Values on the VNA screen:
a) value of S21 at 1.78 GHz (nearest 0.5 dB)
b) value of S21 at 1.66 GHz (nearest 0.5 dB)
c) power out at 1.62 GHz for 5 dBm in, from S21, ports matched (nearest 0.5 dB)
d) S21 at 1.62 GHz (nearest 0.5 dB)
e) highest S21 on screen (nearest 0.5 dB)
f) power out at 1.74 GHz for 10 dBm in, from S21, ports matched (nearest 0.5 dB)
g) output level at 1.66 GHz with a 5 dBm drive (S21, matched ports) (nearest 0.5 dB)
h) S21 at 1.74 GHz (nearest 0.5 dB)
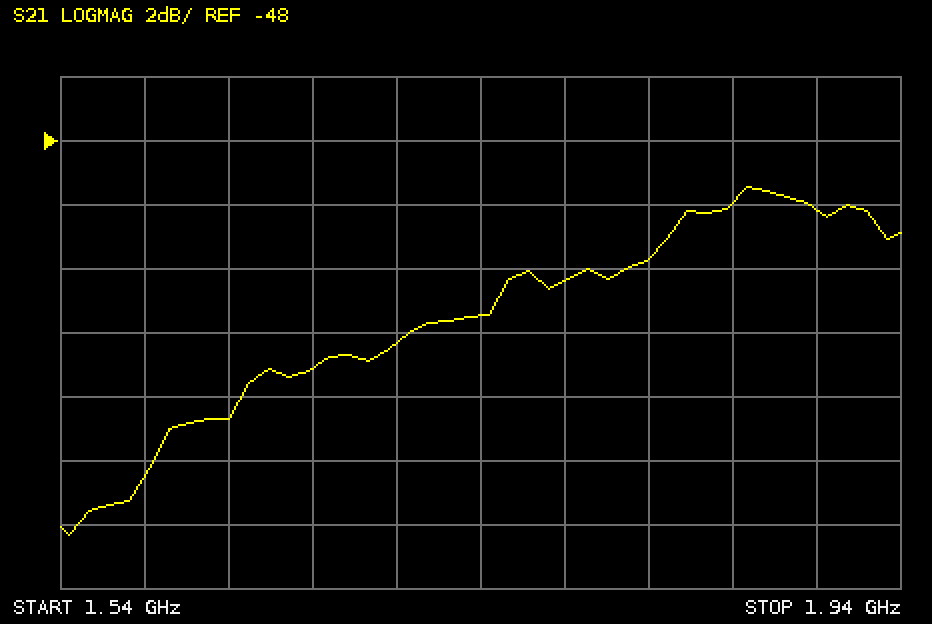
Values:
-52.5 dB
-55.0 dB
-51.5 dBm
-56.5 dB
-49.5 dB
-43.5 dBm
-50.0 dBm
-53.5 dB
